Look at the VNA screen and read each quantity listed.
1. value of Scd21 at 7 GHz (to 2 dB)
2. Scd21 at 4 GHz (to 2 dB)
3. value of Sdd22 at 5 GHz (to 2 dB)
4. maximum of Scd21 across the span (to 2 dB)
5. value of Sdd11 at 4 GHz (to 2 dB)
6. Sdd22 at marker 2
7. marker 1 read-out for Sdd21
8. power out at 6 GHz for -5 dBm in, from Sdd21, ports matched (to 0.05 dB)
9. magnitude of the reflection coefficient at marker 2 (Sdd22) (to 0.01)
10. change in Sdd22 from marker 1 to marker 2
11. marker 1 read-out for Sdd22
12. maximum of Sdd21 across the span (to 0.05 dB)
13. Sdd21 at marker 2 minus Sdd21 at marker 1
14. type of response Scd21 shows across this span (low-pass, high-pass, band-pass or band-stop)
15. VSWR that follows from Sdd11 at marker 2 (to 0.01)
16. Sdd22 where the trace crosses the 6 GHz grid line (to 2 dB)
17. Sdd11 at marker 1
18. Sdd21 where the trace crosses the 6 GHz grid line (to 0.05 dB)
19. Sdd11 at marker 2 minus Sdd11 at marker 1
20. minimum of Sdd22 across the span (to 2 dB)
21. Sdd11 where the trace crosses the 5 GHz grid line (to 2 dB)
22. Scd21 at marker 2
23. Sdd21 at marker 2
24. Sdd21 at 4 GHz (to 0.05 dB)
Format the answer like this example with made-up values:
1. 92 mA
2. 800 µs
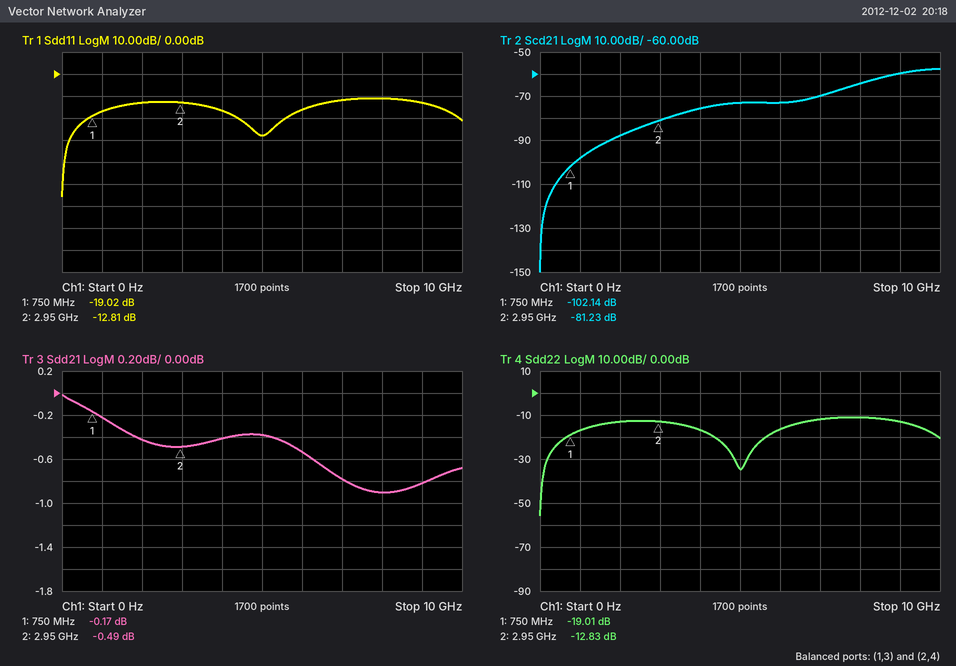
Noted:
1. -70 dB
2. -76 dB
3. -34 dB
4. -58 dB
5. -16 dB
6. -12.83 dB
7. -0.17 dB
8. -5.55 dBm
9. 0.23
10. 6.18 dB
11. -19.01 dB
12. 0.00 dB
13. -0.32 dB
14. high-pass
15. 1.59
16. -16 dB
17. -19.02 dB
18. -0.55 dB
19. 6.21 dB
20. -56 dB
21. -28 dB
22. -81.23 dB
23. -0.49 dB
24. -0.40 dB
